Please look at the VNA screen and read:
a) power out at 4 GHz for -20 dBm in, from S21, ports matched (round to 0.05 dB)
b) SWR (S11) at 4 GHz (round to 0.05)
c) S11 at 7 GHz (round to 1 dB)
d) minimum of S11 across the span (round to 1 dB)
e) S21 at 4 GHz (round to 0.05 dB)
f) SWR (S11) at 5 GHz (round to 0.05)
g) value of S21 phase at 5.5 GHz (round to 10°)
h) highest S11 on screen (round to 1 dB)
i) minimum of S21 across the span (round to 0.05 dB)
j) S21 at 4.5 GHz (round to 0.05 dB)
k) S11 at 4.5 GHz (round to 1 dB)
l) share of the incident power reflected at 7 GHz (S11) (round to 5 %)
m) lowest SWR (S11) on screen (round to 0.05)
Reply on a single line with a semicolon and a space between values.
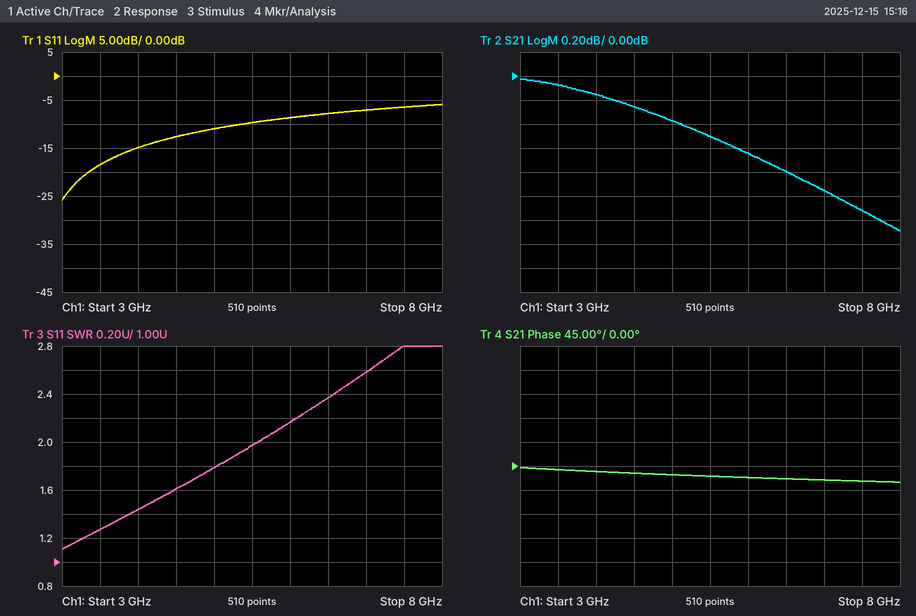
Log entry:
-20.15 dBm; 1.45; -7 dB; -26 dB; -0.15 dB; 1.80; -20°; -6 dB; -1.30 dB; -0.25 dB; -13 dB; 20 %; 1.10
